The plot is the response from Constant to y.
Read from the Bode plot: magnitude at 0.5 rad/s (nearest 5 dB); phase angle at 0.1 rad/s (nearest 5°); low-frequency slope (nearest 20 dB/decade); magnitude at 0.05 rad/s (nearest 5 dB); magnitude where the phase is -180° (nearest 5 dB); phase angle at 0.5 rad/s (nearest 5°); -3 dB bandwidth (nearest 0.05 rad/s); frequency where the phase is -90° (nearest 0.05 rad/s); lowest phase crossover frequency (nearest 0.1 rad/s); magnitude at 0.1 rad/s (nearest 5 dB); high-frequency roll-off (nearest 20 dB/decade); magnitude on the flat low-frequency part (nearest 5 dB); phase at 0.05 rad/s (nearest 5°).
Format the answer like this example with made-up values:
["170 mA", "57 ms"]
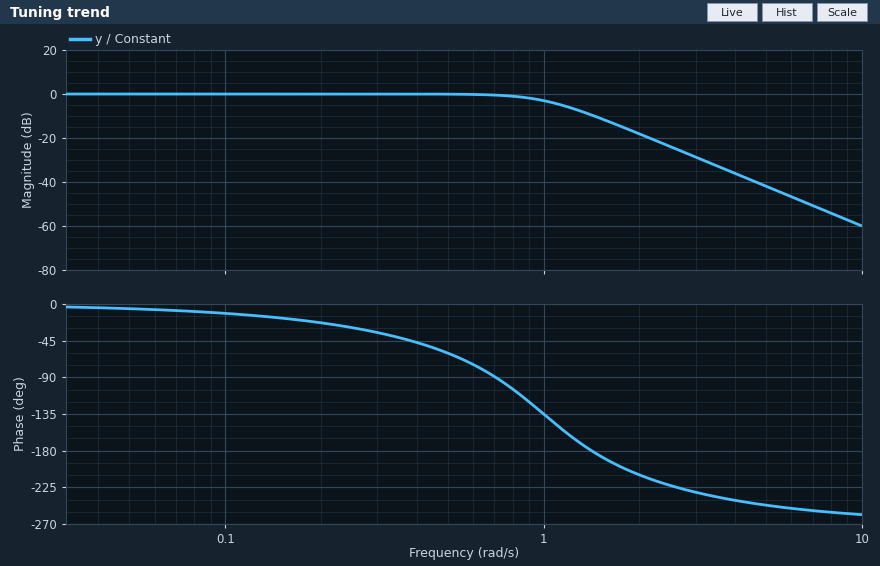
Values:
["0 dB", "-10°", "0 dB/decade", "0 dB", "-10 dB", "-60°", "1.00 rad/s", "0.70 rad/s", "1.4 rad/s", "0 dB", "-60 dB/decade", "0 dB", "-5°"]
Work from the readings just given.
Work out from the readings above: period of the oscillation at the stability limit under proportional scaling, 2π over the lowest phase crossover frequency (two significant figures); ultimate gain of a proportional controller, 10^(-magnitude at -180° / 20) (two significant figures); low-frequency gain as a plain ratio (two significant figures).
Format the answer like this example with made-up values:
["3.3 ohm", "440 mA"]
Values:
["4.5 s", "3.2", "1.0"]
